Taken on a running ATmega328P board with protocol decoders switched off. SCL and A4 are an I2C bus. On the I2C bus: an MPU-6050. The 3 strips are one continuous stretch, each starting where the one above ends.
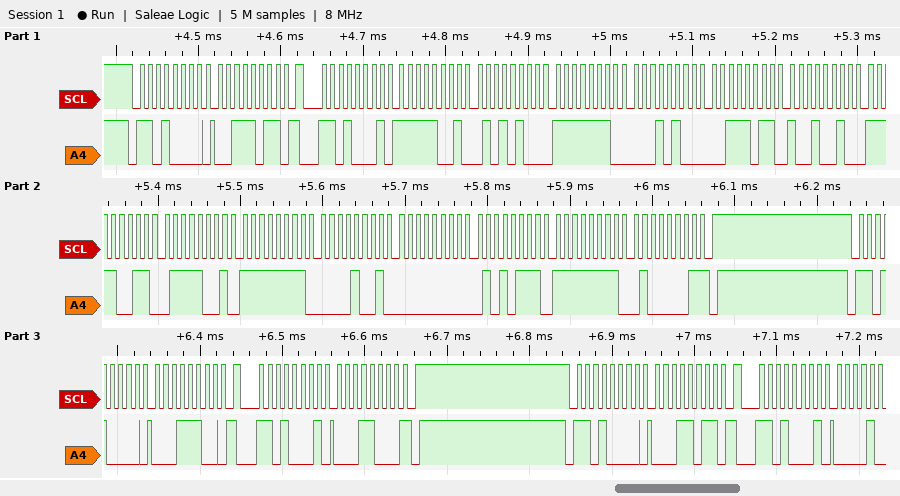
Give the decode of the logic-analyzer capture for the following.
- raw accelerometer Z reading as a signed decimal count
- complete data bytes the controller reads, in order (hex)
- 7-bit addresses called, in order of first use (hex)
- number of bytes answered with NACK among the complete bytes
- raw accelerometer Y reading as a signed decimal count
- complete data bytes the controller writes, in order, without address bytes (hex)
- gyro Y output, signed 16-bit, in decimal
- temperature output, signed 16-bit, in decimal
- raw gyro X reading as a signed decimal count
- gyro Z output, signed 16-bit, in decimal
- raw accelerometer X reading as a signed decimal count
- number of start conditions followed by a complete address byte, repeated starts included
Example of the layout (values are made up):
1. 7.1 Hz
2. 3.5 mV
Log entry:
1. 15250
2. F9 54 FE 14 3B 92 F3 79 FF 09 00 57 FF 41 18
3. 0x68
4. 2
5. -492
6. 3B 1C 1B
7. 87
8. -3207
9. -247
10. -191
11. -1708
12. 6
